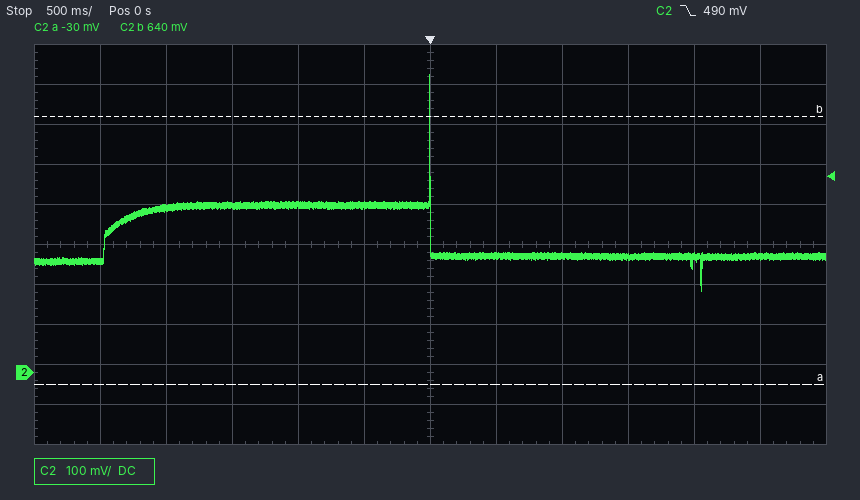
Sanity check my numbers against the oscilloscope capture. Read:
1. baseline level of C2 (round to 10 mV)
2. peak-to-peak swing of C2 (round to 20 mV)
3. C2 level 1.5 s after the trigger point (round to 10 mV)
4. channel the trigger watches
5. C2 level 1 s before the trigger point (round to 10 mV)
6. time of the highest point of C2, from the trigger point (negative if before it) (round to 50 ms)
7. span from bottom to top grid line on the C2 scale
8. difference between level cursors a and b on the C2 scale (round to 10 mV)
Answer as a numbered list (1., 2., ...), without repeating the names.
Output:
1. 290 mV
2. 540 mV
3. 290 mV
4. C2
5. 420 mV
6. 0 ms
7. 1 V
8. 670 mV
